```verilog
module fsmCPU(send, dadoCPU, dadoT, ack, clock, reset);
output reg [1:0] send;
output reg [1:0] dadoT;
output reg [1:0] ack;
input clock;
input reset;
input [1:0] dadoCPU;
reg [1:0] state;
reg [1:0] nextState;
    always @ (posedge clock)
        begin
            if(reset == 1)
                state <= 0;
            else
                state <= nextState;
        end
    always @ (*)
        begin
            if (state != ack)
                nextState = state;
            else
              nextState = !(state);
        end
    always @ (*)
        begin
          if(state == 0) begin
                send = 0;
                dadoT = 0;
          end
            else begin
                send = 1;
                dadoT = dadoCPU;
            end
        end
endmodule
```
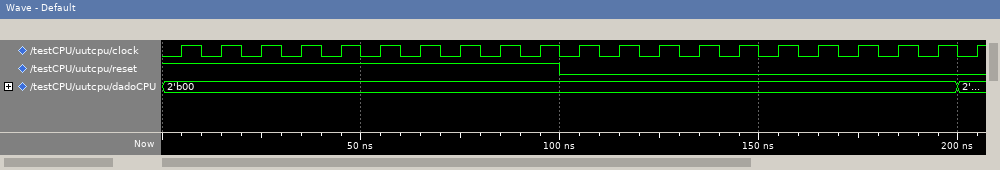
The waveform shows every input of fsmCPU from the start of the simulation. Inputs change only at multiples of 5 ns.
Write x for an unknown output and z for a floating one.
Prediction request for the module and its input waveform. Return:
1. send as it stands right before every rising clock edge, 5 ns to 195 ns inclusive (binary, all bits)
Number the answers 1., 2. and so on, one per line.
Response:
1. 01, 00, 00, 00, 00, 00, 00, 00, 00, 00, 00, 01, 00, 01, 00, 01, 00, 01, 00, 01
